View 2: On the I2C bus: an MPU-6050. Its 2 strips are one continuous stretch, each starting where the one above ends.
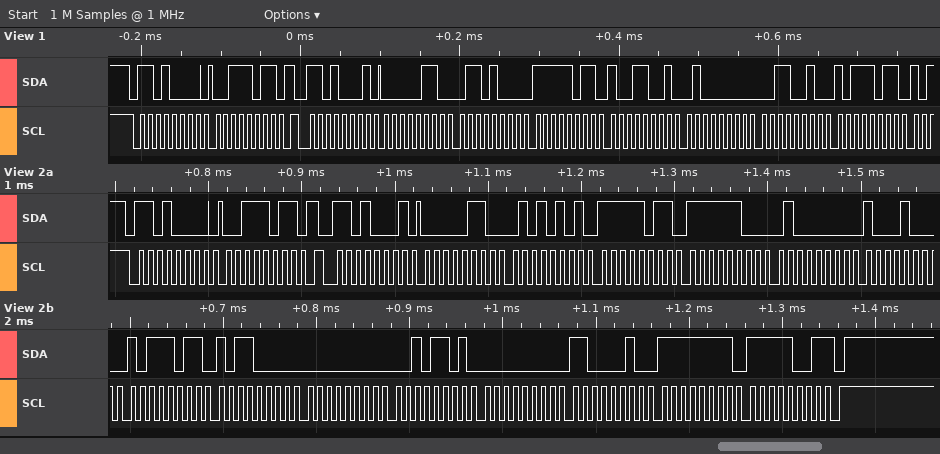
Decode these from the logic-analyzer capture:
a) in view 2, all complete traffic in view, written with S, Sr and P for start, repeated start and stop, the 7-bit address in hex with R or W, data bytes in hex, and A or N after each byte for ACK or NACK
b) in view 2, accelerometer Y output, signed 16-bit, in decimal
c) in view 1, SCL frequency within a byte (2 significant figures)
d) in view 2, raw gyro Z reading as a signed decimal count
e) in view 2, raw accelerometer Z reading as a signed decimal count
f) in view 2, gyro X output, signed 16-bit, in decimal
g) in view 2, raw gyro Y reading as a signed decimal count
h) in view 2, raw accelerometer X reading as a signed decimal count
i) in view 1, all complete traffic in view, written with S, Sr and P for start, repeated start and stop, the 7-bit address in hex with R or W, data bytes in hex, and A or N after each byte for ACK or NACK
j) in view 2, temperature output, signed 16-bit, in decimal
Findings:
S 68W A 3B A Sr 68R A 06 A 55 A FB A FC A 40 A 88 A BB A B0 A 00 A 2D A 00 A C2 A FF A F9 N P
-1028
100 kHz
-7
16520
45
194
1621
S 68W A 3B A Sr 68R A 06 A 68 A FB A 99 A 40 A 32 A BB A
-17488
